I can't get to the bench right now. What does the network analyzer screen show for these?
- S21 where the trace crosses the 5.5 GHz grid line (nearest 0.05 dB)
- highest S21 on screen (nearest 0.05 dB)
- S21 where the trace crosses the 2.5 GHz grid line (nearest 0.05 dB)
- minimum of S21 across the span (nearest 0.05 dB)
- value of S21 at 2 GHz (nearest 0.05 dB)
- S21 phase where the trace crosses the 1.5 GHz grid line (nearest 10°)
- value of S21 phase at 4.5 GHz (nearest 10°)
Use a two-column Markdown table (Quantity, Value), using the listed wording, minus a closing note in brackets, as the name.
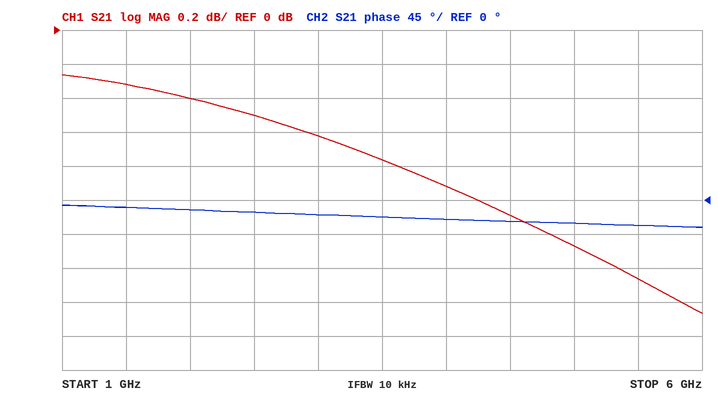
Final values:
| Quantity | Value |
|---|---|
| S21 where the trace crosses the 5.5 GHz grid line | -1.45 dB |
| highest S21 on screen | -0.25 dB |
| S21 where the trace crosses the 2.5 GHz grid line | -0.50 dB |
| minimum of S21 across the span | -1.65 dB |
| value of S21 at 2 GHz | -0.40 dB |
| S21 phase where the trace crosses the 1.5 GHz grid line | -10° |
| value of S21 phase at 4.5 GHz | -30° |
